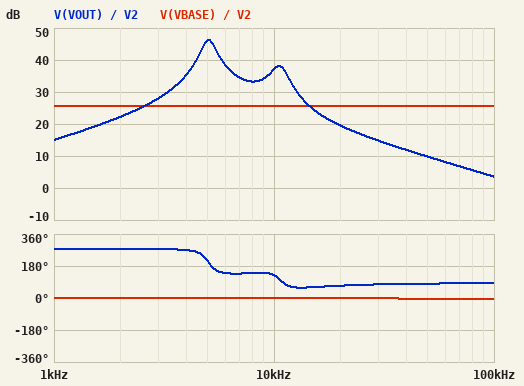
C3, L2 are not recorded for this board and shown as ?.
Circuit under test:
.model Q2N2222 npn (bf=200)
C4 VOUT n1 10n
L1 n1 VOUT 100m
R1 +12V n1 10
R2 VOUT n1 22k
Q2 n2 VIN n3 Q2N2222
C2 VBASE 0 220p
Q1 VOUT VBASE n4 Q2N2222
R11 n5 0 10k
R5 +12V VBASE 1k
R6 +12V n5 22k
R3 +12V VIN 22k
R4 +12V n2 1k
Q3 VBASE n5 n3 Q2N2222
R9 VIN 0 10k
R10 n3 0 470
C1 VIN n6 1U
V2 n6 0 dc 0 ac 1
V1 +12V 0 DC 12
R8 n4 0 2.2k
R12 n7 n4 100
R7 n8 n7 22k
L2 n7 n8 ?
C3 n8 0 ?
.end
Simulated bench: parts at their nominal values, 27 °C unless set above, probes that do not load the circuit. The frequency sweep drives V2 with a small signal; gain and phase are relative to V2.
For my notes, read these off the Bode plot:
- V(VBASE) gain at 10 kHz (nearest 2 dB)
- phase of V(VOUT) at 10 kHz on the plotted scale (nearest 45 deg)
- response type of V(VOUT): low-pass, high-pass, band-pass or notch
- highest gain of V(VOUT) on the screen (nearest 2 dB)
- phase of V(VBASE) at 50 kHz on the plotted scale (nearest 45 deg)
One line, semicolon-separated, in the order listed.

26 dB; 135 deg; band-pass; 46 dB; 0 deg
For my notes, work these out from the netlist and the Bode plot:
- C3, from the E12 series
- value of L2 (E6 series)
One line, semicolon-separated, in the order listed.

4.7 nF; 47 mH
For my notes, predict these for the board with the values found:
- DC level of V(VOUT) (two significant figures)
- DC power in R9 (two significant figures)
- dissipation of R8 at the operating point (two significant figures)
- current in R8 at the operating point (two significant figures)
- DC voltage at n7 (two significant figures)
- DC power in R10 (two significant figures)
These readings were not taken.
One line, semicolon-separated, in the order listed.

12 V; 1.3 mW; 30 mW; 3.7 mA; 8.2 V; 17 mW
